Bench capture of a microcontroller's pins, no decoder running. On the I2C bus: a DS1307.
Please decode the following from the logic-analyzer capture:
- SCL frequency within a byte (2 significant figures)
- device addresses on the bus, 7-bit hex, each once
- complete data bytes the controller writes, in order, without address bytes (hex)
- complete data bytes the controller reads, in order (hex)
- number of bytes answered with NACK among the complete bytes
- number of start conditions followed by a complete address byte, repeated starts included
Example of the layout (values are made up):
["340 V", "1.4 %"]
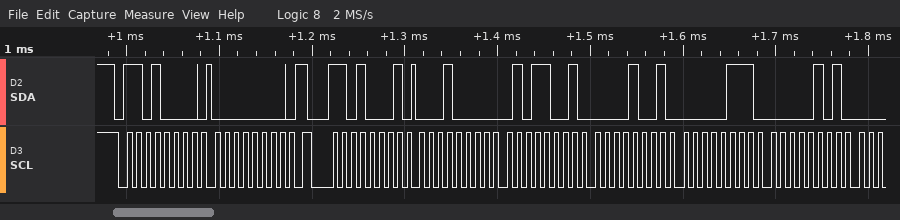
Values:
["100 kHz", "0x68", "00", "10 59 09 07 05", "0", "2"]
